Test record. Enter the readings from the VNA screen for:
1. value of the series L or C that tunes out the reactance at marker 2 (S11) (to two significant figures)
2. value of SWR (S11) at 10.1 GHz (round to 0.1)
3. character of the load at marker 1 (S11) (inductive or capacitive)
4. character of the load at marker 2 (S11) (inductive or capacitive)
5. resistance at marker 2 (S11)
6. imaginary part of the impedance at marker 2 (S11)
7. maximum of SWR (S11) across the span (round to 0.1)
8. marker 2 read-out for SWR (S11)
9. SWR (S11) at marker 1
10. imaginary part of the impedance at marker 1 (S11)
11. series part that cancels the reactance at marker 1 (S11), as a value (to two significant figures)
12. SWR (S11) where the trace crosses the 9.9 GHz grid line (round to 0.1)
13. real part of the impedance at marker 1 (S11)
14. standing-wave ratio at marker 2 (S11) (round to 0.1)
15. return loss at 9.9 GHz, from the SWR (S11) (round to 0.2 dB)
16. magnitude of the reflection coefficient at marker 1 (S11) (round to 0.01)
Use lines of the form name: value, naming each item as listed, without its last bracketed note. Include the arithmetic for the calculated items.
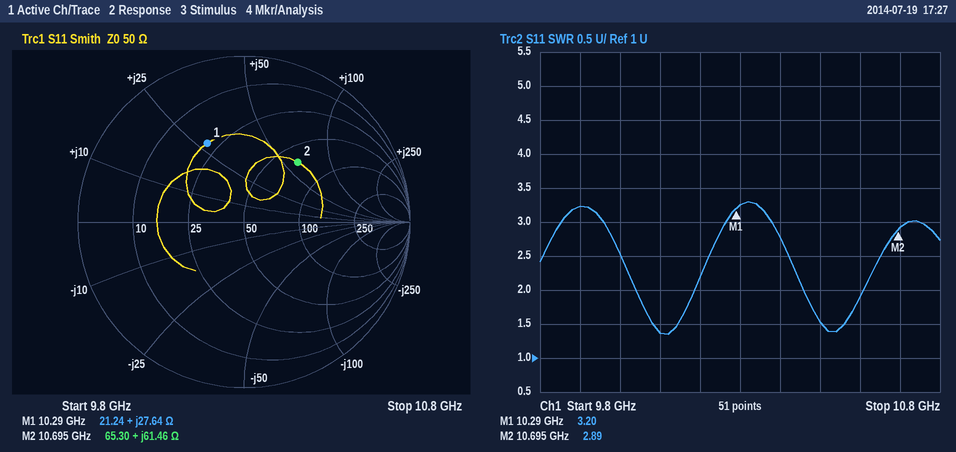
value of the series L or C that tunes out the reactance at marker 2 (S11): C = 1/(2π × 10.695 GHz × 61.46 Ω) ≈ 242 fF, so 240 fF to two significant figures
value of SWR (S11) at 10.1 GHz: 1.4
character of the load at marker 1 (S11): inductive
character of the load at marker 2 (S11): inductive
resistance at marker 2: 65.30 Ω
imaginary part of the impedance at marker 2: +61.46 Ω
maximum of SWR (S11) across the span: 3.3
marker 2 read-out for SWR: 2.89
SWR (S11) at marker 1: 3.20
imaginary part of the impedance at marker 1: +27.64 Ω
series part that cancels the reactance at marker 1 (S11), as a value: C = 1/(2π × 10.29 GHz × 27.64 Ω) ≈ 560 fF
SWR (S11) where the trace crosses the 9.9 GHz grid line: 3.2
real part of the impedance at marker 1: 21.24 Ω
standing-wave ratio at marker 2 (S11): 2.9
return loss at 9.9 GHz, from the SWR (S11): −20 log10((3.2 − 1)/(3.2 + 1)) ≈ 5.6 dB
magnitude of the reflection coefficient at marker 1 (S11): 0.52
